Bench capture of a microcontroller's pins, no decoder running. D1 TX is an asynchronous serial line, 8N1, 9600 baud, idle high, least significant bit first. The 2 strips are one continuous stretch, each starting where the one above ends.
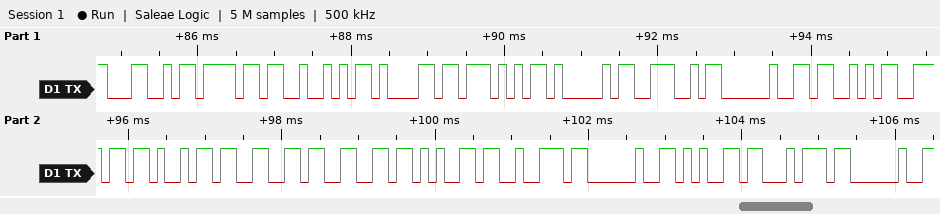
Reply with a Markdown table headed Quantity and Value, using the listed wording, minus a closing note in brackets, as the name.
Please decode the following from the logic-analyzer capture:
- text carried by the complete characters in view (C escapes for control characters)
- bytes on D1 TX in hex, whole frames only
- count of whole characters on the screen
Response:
| Quantity | Value |
|---|---|
| text carried by the complete characters in view | "LoRaWAN Sniffer et " |
| bytes on D1 TX in hex, whole frames only | 4C 6F 52 61 57 41 4E 20 53 6E 69 66 66 65 72 20 65 74 20 |
| count of whole characters on the screen | 19 |
